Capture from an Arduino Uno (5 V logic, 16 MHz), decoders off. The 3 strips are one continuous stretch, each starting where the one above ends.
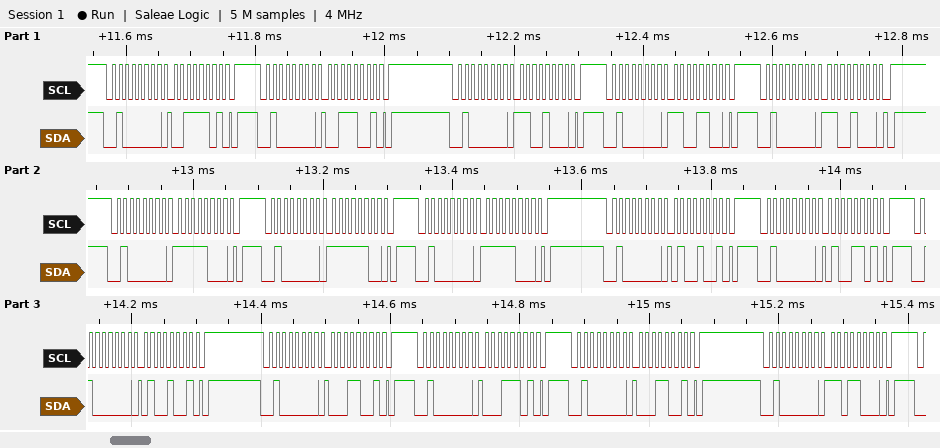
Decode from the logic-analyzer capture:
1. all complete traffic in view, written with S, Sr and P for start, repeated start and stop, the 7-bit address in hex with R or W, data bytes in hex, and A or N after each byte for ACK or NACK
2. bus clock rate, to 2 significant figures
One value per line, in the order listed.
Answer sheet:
S 20W A 3D A P S 20W A 39 A P S 20W A C8 A P S 20W A CC A P S 20W A C8 A P S 20W A F8 A P S 20W A FC A P S 20W A F8 A P S 20W A 49 A P S 20W A 4D A P S 20W A 49 A P S 20W A 19 A P S 20W A 1D A P S 20W A 19 A P S 20W A D8 A P
100 kHz
